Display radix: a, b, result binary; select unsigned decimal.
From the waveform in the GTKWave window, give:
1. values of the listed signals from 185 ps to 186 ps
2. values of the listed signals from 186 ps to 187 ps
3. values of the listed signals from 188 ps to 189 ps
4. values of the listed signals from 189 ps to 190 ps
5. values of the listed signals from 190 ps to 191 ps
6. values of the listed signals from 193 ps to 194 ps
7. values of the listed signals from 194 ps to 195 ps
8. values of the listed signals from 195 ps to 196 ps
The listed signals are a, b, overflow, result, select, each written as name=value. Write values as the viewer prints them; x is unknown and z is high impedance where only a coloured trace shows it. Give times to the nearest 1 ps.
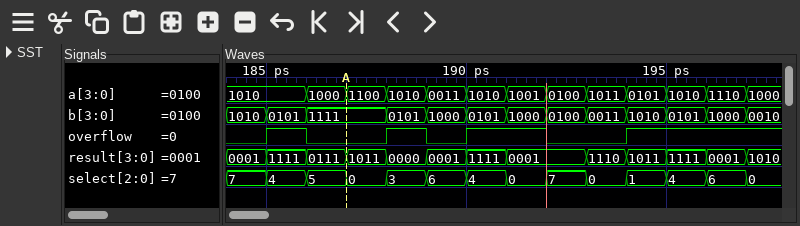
a=1010, b=0101, overflow=1, result=1111, select=4
a=1000, b=1111, overflow=0, result=0111, select=5
a=1010, b=0101, overflow=1, result=0000, select=3
a=0011, b=1000, overflow=0, result=0001, select=6
a=1010, b=0101, overflow=1, result=1111, select=4
a=1011, b=0011, overflow=0, result=1110, select=0
a=0101, b=1010, overflow=1, result=1011, select=1
a=1010, b=0101, overflow=1, result=1111, select=4
